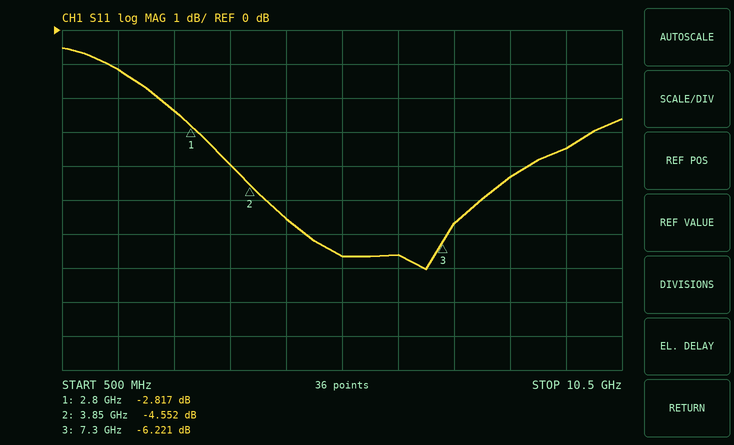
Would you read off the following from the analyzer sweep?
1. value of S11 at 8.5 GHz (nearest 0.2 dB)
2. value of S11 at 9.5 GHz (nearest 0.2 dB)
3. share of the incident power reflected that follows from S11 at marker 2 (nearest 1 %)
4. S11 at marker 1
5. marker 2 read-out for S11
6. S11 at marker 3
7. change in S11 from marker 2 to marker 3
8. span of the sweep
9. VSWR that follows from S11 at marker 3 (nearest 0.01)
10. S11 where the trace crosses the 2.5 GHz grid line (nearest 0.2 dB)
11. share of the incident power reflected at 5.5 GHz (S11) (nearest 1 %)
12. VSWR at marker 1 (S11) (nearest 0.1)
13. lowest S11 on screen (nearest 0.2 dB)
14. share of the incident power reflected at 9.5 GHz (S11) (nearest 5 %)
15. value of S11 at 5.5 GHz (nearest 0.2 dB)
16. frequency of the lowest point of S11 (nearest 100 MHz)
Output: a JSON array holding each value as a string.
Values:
["-4.4 dB", "-3.4 dB", "35 %", "-2.817 dB", "-4.552 dB", "-6.221 dB", "-1.669 dB", "10 GHz", "2.91", "-2.4 dB", "22 %", "6.2", "-7.0 dB", "45 %", "-6.6 dB", "7.0 GHz"]
